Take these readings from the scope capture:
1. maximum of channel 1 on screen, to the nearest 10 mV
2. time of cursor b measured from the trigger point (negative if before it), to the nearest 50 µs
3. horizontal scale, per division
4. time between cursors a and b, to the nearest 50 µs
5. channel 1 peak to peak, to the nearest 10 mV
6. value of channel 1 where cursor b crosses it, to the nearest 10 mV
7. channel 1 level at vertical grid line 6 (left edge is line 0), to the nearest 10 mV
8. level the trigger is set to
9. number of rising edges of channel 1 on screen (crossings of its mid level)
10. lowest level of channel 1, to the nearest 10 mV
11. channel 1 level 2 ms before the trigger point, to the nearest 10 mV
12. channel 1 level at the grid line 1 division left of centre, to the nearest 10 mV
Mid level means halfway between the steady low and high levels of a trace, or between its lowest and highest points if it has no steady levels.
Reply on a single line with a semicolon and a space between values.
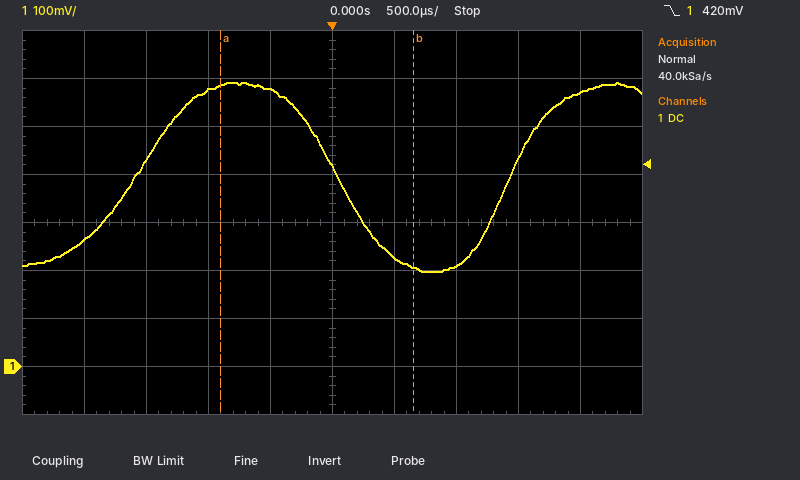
590 mV; +650 µs; 500 µs; 1.55 ms; 390 mV; 210 mV; 230 mV; 420 mV; 2; 200 mV; 260 mV; 580 mV
